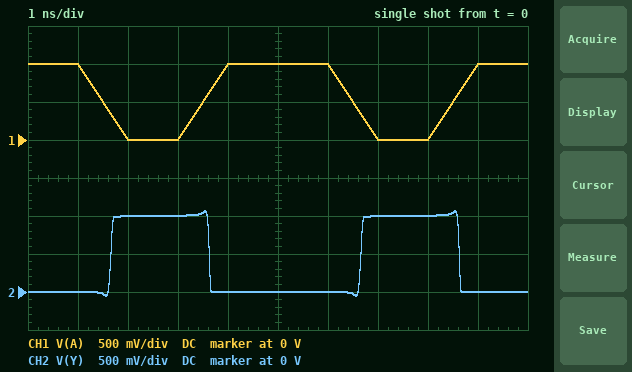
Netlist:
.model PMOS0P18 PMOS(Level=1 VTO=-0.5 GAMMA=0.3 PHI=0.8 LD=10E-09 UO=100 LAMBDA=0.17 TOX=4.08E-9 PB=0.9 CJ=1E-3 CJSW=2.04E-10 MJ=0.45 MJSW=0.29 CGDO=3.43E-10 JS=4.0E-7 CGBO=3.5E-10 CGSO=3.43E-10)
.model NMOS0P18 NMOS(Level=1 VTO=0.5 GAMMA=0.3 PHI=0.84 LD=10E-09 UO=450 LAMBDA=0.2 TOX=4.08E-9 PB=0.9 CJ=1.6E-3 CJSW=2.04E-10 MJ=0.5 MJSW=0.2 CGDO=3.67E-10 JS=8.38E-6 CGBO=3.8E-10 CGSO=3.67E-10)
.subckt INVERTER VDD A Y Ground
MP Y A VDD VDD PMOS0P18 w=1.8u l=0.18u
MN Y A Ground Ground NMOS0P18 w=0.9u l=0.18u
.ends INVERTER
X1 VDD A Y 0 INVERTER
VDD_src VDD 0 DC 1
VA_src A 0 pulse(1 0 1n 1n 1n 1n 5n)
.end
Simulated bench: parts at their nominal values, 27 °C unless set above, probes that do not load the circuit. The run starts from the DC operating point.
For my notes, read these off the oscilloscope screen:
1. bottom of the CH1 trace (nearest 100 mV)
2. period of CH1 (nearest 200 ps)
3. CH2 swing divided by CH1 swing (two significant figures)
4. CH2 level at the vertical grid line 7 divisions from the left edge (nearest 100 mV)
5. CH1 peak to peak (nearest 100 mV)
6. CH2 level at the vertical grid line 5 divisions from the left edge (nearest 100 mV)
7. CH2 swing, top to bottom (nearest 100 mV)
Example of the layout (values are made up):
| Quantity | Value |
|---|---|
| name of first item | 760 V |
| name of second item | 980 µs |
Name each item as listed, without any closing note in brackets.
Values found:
| Quantity | Value |
|---|---|
| bottom of the CH1 trace | 0 V |
| period of CH1 | 5.0 ns |
| CH2 swing divided by CH1 swing | 1.1 |
| CH2 level at the vertical grid line 7 divisions from the left edge | 1.0 V |
| CH1 peak to peak | 1.0 V |
| CH2 level at the vertical grid line 5 divisions from the left edge | 0 V |
| CH2 swing, top to bottom | 1.1 V |
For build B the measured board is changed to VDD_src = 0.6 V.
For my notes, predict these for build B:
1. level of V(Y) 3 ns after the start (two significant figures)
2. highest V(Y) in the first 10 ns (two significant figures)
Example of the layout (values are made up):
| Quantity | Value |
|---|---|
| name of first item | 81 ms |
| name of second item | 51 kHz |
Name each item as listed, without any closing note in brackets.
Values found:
| Quantity | Value |
|---|---|
| level of V(Y) 3 ns after the start | 600 mV |
| highest V(Y) in the first 10 ns | 990 mV |
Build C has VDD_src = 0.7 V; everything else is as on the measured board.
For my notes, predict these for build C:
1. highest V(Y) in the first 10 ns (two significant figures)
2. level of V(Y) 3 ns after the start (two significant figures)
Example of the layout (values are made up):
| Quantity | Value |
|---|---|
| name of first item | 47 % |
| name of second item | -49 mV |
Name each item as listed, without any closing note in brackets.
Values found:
| Quantity | Value |
|---|---|
| highest V(Y) in the first 10 ns | 1.0 V |
| level of V(Y) 3 ns after the start | 700 mV |
